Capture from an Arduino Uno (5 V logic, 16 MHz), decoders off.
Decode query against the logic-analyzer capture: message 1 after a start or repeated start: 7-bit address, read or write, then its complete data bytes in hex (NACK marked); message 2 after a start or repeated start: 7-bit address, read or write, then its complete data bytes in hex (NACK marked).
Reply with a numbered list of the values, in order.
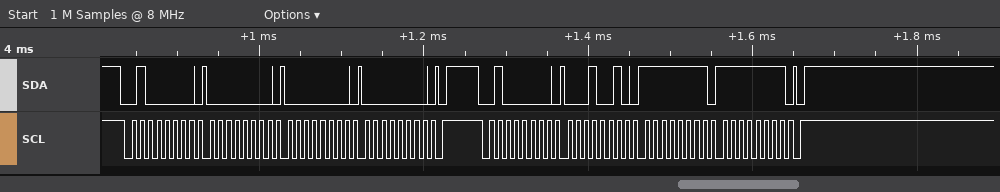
1. 0x20 write: 00 00 00
2. 0x20 write: 12 FF FF
